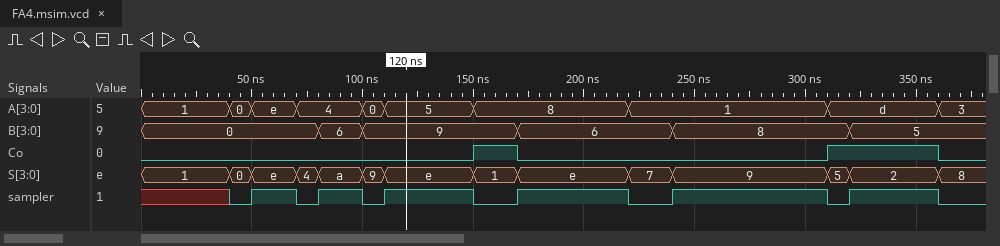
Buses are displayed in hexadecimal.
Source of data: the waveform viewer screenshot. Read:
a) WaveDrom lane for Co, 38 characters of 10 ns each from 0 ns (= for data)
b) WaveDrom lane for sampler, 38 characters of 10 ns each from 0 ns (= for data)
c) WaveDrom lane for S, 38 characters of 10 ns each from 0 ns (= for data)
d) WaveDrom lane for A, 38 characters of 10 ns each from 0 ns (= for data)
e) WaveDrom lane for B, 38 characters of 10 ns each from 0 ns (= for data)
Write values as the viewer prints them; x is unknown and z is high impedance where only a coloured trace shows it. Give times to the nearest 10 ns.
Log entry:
{name: 'Co', wave: '0..............1.0.............1....0.'}
{name: 'sampler', wave: 'x...01.01.01...0.1....0.1......01...0.'}
{name: 'S', wave: '=...==.==.==...=.=....=.=......==...=.', data: '1 0 e 4 a 9 e 1 e 7 9 5 2 8'}
{name: 'A', wave: '=...==.=..==...=......=........=....=.', data: '1 0 e 4 0 5 8 1 d 3'}
{name: 'B', wave: '=.......=.=......=......=.......=.....', data: '0 6 9 6 8 5'}
